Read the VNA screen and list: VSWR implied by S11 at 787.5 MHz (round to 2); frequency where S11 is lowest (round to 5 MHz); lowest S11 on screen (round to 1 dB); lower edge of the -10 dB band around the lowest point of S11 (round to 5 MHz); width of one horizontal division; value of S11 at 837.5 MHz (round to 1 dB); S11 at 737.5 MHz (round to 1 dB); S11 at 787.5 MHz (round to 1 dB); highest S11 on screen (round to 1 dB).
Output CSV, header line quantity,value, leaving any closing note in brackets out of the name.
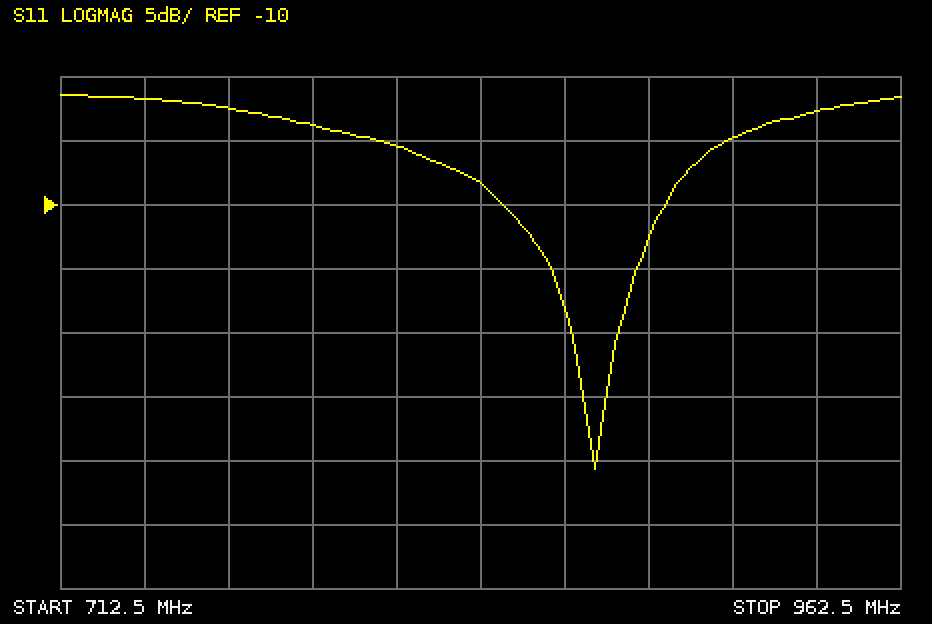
quantity,value
VSWR implied by S11 at 787.5 MHz,4
frequency where S11 is lowest,870 MHz
lowest S11 on screen,-31 dB
lower edge of the -10 dB band around the lowest point of S11,845 MHz
width of one horizontal division,25 MHz
value of S11 at 837.5 MHz,-8 dB
S11 at 737.5 MHz,-2 dB
S11 at 787.5 MHz,-4 dB
highest S11 on screen,-1 dB
